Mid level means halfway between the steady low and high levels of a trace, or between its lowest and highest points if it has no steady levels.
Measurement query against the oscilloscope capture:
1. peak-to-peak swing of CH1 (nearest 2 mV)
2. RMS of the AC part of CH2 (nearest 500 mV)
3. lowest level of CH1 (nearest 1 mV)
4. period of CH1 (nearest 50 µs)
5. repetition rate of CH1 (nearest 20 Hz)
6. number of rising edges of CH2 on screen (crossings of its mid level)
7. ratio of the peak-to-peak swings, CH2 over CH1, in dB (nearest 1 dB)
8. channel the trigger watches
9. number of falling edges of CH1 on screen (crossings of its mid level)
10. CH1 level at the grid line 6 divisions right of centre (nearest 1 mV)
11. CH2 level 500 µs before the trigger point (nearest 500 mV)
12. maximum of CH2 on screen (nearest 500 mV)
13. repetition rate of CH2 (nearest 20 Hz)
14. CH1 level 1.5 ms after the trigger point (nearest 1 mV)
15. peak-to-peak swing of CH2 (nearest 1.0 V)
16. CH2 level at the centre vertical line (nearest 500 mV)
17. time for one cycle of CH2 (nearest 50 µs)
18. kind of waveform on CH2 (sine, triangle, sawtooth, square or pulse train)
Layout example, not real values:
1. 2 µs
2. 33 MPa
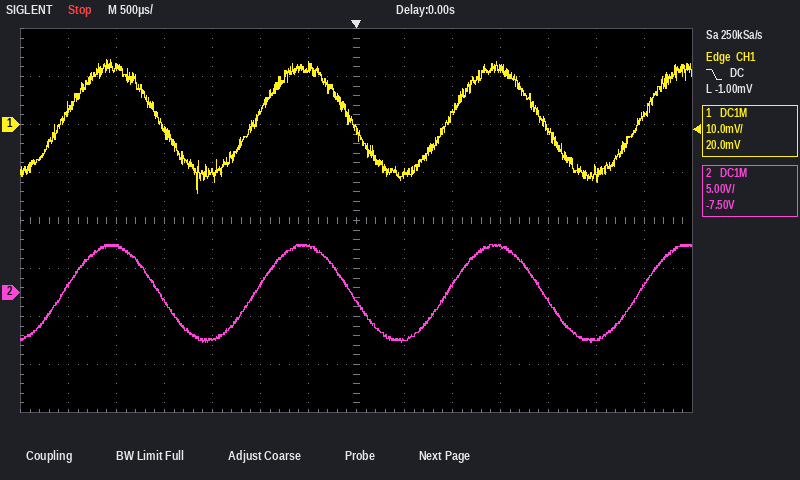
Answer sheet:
1. 28 mV
2. 3.5 V
3. -14 mV
4. 2.00 ms
5. 500 Hz
6. 4
7. 51 dB
8. CH1
9. 3
10. 2 mV
11. 5.0 V
12. 5.0 V
13. 500 Hz
14. 12 mV
15. 10.0 V
16. -1.0 V
17. 2.00 ms
18. sine
